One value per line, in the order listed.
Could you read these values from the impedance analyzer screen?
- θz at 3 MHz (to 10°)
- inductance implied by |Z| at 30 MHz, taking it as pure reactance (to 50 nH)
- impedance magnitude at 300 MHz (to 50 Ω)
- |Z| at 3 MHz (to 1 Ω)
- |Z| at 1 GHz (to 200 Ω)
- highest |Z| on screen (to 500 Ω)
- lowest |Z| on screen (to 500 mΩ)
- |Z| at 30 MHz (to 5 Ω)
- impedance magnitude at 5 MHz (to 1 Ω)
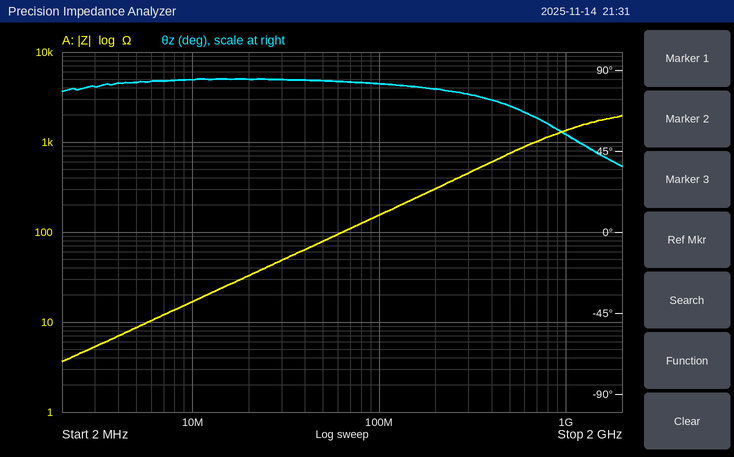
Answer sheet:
80°
250 nH
450 Ω
5 Ω
1.4 kΩ
2.0 kΩ
3.5 Ω
50 Ω
9 Ω
